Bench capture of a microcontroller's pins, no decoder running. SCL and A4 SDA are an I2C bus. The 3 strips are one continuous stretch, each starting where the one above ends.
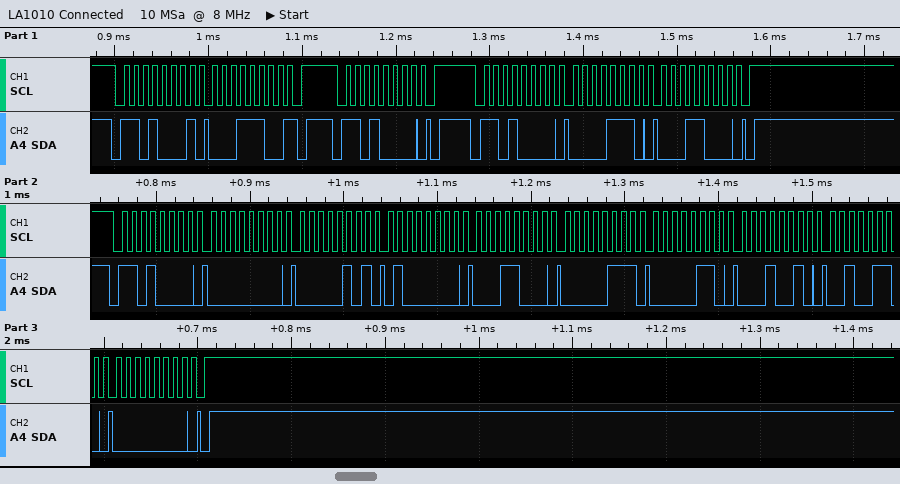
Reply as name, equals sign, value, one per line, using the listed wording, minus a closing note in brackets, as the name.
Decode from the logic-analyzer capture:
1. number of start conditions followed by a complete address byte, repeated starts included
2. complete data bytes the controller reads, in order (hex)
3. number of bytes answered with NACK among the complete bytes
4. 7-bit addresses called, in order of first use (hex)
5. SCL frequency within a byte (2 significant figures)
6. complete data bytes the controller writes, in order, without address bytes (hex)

number of start conditions followed by a complete address byte, repeated starts included = 4
complete data bytes the controller reads, in order = 1C
number of bytes answered with NACK among the complete bytes = 1
7-bit addresses called, in order of first use = 0x68
SCL frequency within a byte = 100 kHz
complete data bytes the controller writes, in order, without address bytes = 0E 18 00 05 40 18 07 06 12 26 00
